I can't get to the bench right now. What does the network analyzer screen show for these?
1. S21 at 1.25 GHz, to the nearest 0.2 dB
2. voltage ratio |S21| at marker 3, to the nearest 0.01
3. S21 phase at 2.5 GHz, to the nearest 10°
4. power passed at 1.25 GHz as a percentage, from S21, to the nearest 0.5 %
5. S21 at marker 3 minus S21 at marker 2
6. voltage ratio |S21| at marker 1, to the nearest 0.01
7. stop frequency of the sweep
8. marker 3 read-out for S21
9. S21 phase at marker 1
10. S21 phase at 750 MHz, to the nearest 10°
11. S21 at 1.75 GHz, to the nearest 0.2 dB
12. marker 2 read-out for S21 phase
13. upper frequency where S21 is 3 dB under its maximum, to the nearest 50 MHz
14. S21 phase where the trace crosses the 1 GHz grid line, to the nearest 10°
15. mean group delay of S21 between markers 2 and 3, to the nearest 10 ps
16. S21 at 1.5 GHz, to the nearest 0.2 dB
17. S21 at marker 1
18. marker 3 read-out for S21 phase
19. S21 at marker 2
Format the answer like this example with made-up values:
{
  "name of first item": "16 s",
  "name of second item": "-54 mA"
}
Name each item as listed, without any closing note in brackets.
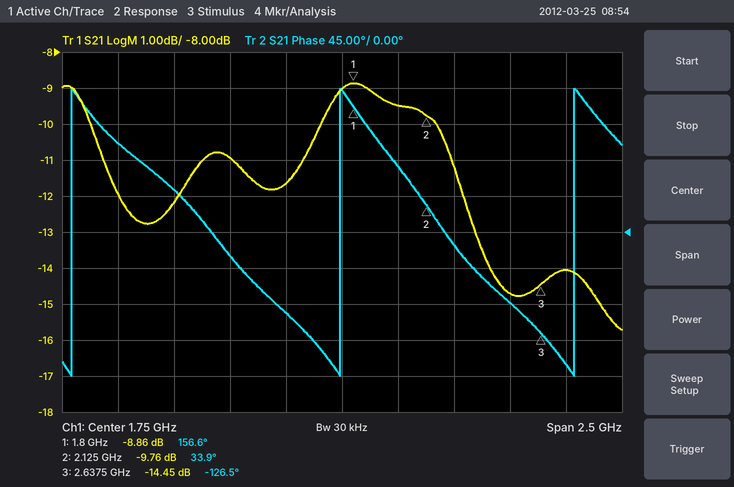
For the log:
{
  "S21 at 1.25 GHz, to the nearest 0.2 dB": "-11.0 dB",
  "voltage ratio |S21| at marker 3, to the nearest 0.01": "0.19",
  "S21 phase at 2.5 GHz, to the nearest 10°": "-90°",
  "power passed at 1.25 GHz as a percentage, from S21, to the nearest 0.5 %": "8.0 %",
  "S21 at marker 3 minus S21 at marker 2": "-4.69 dB",
  "voltage ratio |S21| at marker 1, to the nearest 0.01": "0.36",
  "stop frequency of the sweep": "3 GHz",
  "marker 3 read-out for S21": "-14.45 dB",
  "S21 phase at marker 1": "156.6°",
  "S21 phase at 750 MHz, to the nearest 10°": "110°",
  "S21 at 1.75 GHz, to the nearest 0.2 dB": "-9.0 dB",
  "marker 2 read-out for S21 phase": "33.9°",
  "upper frequency where S21 is 3 dB under its maximum, to the nearest 50 MHz": "2.30 GHz",
  "S21 phase where the trace crosses the 1 GHz grid line, to the nearest 10°": "50°",
  "mean group delay of S21 between markers 2 and 3, to the nearest 10 ps": "870 ps",
  "S21 at 1.5 GHz, to the nearest 0.2 dB": "-11.6 dB",
  "S21 at marker 1": "-8.86 dB",
  "marker 3 read-out for S21 phase": "-126.5°",
  "S21 at marker 2": "-9.76 dB"
}
